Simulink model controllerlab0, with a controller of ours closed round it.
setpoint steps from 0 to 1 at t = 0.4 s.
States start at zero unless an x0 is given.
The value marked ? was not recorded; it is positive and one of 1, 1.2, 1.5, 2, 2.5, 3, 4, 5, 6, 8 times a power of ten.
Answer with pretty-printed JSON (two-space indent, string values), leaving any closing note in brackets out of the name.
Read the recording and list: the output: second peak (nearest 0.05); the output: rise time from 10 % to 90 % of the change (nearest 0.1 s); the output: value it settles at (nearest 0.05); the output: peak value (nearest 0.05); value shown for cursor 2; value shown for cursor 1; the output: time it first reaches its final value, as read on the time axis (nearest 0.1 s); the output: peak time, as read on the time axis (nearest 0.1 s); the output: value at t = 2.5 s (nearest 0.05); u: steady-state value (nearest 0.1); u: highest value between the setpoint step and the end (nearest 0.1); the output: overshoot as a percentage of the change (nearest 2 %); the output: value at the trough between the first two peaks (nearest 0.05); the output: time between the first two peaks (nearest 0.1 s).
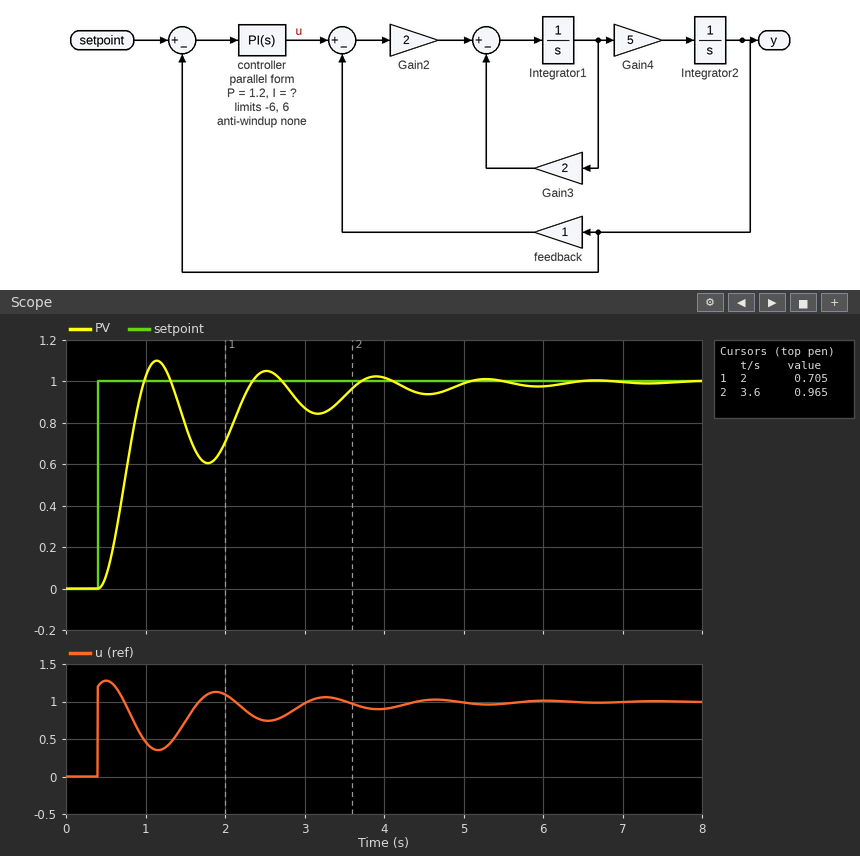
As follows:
{
  "the output: second peak": "1.05",
  "the output: rise time from 10 % to 90 % of the change": "0.4 s",
  "the output: value it settles at": "1.00",
  "the output: peak value": "1.10",
  "value shown for cursor 2": "0.965",
  "value shown for cursor 1": "0.705",
  "the output: time it first reaches its final value, as read on the time axis": "1.0 s",
  "the output: peak time, as read on the time axis": "1.1 s",
  "the output: value at t = 2.5 s": "1.05",
  "u: steady-state value": "1.0",
  "u: highest value between the setpoint step and the end": "1.3",
  "the output: overshoot as a percentage of the change": "10 %",
  "the output: value at the trough between the first two peaks": "0.60",
  "the output: time between the first two peaks": "1.4 s"
}
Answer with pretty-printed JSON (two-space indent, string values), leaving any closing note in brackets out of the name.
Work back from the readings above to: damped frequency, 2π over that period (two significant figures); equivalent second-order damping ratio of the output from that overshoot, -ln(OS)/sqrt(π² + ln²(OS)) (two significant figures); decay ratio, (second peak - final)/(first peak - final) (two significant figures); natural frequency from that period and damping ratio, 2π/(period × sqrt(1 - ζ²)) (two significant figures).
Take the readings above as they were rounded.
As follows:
{
  "damped frequency, 2π over that period": "4.5 rad/s",
  "equivalent second-order damping ratio of the output from that overshoot, -ln(OS)/sqrt(π² + ln²(OS))": "0.59",
  "decay ratio, (second peak - final)/(first peak - final)": "0.50",
  "natural frequency from that period and damping ratio, 2π/(period × sqrt(1 - ζ²))": "5.6 rad/s"
}
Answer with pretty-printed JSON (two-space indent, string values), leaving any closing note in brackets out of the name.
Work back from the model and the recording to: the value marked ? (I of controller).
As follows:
{
  "the value marked ?": "1.5"
}
